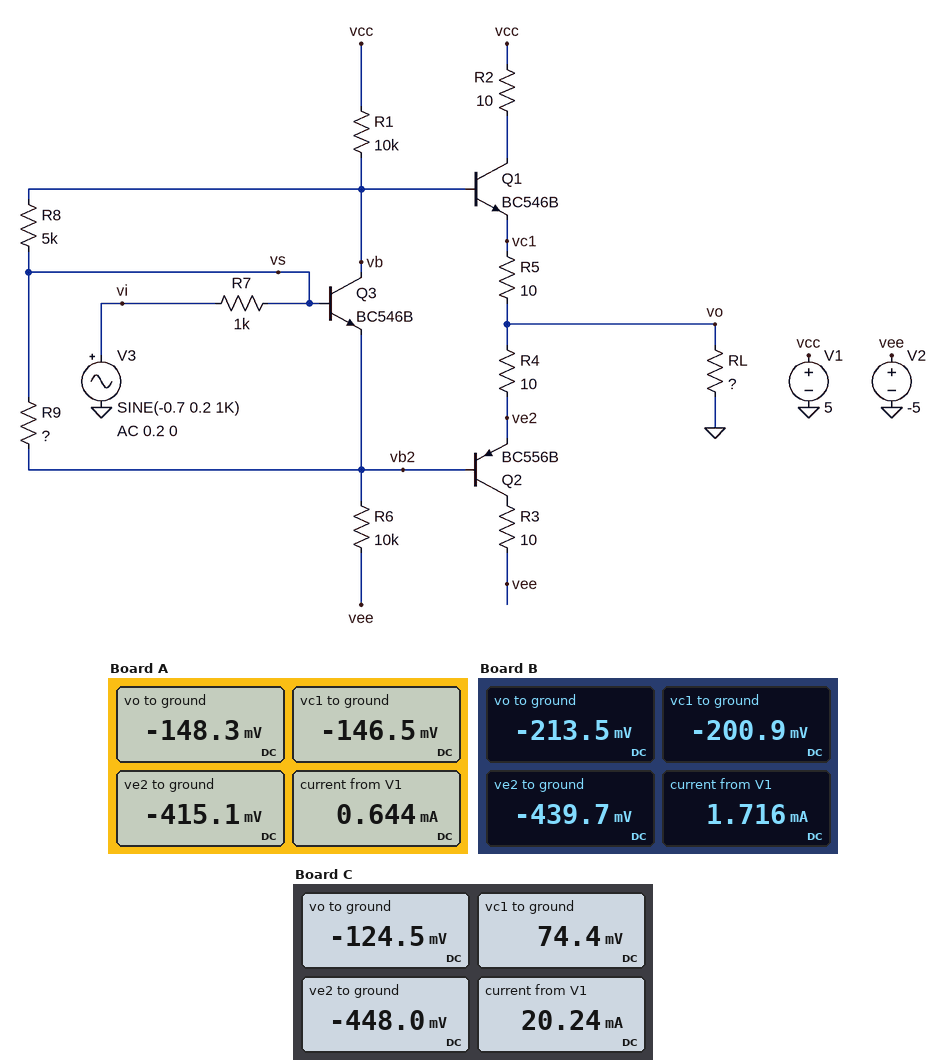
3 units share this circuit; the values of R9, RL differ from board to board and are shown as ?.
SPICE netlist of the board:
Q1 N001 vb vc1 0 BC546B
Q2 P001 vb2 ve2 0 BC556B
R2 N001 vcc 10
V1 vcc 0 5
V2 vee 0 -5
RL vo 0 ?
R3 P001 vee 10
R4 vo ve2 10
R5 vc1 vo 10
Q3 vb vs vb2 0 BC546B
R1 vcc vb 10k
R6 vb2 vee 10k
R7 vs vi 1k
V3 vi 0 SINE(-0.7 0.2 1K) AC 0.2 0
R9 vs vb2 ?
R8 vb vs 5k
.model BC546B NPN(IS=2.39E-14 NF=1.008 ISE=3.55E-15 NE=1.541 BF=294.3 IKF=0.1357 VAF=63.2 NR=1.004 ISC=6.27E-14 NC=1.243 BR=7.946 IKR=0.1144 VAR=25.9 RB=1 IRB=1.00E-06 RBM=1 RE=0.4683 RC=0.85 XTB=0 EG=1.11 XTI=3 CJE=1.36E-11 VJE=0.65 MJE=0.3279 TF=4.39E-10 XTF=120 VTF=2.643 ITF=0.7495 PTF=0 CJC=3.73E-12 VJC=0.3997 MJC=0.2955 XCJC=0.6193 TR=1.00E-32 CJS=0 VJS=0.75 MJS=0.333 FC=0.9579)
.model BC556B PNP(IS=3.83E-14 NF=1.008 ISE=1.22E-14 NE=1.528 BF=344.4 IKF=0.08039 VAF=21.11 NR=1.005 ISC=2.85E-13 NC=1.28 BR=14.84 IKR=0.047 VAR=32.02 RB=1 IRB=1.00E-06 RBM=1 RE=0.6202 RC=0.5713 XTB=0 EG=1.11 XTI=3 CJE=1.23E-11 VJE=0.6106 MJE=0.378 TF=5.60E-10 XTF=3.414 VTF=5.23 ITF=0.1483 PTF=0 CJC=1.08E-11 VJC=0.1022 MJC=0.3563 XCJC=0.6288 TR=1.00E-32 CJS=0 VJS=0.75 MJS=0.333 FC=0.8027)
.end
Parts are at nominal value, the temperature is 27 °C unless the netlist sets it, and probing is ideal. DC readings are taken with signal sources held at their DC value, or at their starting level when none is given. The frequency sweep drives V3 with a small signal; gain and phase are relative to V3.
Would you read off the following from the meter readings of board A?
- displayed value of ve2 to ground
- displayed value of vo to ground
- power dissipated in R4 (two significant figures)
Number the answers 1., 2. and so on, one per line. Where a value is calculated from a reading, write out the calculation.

1. -415.1 mV
2. -148.3 mV
3. (-148.3 mV - (-415.1 mV))^2 / 10 Ω = 7.1 mW
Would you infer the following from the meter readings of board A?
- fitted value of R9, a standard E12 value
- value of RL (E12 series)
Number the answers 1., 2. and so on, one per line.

1. 15 kΩ
2. 5.6 Ω
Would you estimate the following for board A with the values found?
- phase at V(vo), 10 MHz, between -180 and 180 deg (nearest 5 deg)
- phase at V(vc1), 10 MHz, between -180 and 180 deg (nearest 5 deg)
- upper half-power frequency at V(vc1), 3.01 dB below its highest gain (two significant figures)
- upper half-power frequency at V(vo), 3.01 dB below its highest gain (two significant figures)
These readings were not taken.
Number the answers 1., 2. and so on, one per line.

1. -45 deg
2. -45 deg
3. 14 MHz
4. 16 MHz
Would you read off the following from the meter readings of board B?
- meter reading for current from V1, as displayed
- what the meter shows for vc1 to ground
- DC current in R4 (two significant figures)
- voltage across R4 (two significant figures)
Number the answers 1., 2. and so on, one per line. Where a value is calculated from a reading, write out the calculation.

1. 1.716 mA
2. -200.9 mV
3. (-213.5 mV - (-439.7 mV)) / 10 Ω = 23 mA
4. -213.5 mV - (-439.7 mV) = 230 mV
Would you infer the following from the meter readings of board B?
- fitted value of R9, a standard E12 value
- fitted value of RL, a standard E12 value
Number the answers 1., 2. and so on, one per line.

1. 10 kΩ
2. 10 Ω
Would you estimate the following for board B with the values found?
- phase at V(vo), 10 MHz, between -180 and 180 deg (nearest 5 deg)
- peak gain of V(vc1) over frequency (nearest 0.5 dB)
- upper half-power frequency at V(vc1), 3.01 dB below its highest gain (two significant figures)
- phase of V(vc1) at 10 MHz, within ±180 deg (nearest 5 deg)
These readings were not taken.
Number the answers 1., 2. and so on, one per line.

1. -40 deg
2. -16.0 dB
3. 1.4 MHz
4. 0 deg
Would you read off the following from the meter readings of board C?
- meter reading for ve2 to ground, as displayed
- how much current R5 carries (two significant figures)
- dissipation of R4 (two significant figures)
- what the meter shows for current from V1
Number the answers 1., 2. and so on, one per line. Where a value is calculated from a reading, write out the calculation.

1. -448.0 mV
2. (74.4 mV - (-124.5 mV)) / 10 Ω = 20 mA
3. (-124.5 mV - (-448 mV))^2 / 10 Ω = 10 mW
4. 20.24 mA
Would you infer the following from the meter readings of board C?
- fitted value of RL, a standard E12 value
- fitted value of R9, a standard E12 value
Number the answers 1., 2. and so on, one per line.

1. 10 Ω
2. 2.7 kΩ
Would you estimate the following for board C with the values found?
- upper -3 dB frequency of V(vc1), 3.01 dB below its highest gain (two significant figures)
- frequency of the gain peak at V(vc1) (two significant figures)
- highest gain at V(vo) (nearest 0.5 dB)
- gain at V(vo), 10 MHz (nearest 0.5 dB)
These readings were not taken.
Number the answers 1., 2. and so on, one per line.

1. 10 MHz
2. 4.1 MHz
3. -12.5 dB
4. -19.5 dB
